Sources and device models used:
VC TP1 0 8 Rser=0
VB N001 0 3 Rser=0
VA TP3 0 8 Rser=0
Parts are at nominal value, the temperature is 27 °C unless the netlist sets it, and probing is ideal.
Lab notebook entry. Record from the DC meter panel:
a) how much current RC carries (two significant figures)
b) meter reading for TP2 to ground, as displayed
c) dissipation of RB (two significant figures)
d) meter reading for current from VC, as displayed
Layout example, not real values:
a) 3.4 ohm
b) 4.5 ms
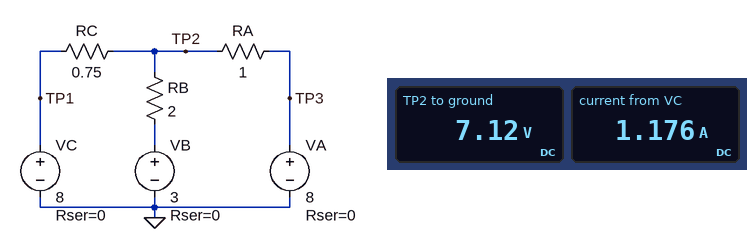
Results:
a) 1.2 A
b) 7.12 V
c) 8.5 W
d) 1.176 A
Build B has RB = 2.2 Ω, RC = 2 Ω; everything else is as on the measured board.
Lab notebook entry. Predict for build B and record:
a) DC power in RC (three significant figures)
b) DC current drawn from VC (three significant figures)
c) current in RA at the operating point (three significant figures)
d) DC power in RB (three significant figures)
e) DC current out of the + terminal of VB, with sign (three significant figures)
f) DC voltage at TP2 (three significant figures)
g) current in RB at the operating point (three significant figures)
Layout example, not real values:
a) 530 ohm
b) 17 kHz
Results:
a) 676 mW
b) 581 mA
c) 1.16 A
d) 6.69 W
e) -1.74 A
f) 6.84 V
g) 1.74 A
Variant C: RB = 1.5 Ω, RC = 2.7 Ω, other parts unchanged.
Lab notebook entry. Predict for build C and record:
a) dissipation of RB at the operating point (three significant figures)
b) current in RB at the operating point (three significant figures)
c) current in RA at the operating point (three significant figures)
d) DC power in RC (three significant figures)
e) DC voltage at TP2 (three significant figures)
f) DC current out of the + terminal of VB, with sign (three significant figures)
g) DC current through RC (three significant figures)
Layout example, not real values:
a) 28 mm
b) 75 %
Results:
a) 7.54 W
b) 2.24 A
c) 1.64 A
d) 992 mW
e) 6.36 V
f) -2.24 A
g) 606 mA
